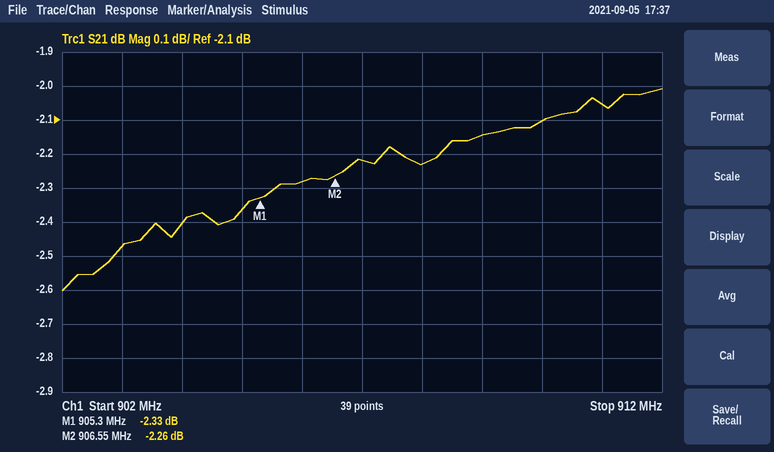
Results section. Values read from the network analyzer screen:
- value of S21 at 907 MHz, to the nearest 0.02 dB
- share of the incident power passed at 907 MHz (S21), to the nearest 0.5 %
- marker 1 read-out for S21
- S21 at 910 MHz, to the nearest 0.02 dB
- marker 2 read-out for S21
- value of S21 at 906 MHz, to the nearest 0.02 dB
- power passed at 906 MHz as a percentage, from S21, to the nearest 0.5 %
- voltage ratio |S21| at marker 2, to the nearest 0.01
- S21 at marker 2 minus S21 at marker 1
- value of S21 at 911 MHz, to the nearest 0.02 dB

-2.22 dB
60.0 %
-2.33 dB
-2.10 dB
-2.26 dB
-2.28 dB
59.0 %
0.77
0.07 dB
-2.06 dB
